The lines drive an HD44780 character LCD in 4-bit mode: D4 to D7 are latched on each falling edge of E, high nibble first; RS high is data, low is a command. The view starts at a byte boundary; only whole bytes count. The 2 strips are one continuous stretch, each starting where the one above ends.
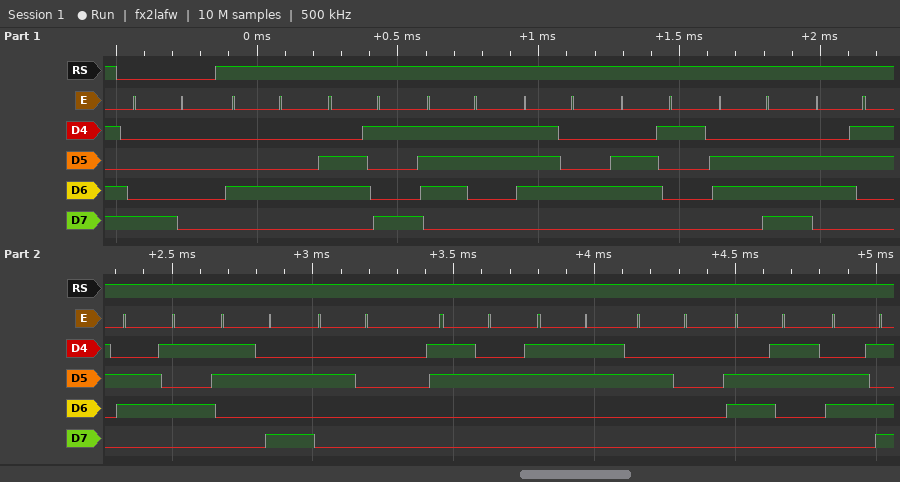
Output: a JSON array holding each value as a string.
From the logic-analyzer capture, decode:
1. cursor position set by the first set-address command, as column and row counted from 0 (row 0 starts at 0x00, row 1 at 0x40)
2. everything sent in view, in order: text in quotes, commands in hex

["column 0, row 0", "0x80 \"Distance: 23 cm\""]
